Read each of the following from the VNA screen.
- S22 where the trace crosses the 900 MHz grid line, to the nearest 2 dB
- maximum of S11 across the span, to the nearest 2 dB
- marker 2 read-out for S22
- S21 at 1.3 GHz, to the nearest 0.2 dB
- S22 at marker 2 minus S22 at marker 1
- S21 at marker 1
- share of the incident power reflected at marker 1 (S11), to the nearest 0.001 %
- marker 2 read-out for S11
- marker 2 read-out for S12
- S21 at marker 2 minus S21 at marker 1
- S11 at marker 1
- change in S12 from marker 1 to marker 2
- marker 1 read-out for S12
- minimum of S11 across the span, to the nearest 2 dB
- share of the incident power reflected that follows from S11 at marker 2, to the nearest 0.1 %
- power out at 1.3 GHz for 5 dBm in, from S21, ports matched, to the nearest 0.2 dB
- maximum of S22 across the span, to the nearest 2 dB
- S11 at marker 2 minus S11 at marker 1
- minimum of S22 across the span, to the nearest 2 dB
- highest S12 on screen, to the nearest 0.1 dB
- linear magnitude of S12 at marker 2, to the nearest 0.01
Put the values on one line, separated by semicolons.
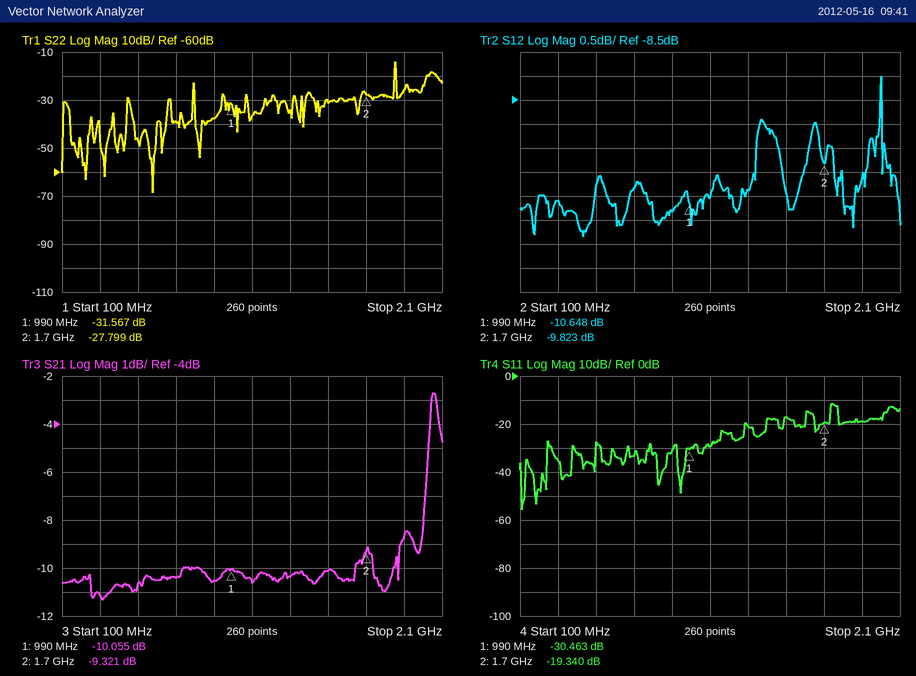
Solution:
-38 dB; -12 dB; -27.799 dB; -10.4 dB; 3.768 dB; -10.055 dB; 0.090 %; -19.340 dB; -9.823 dB; 0.734 dB; -30.463 dB; 0.825 dB; -10.648 dB; -56 dB; 1.2 %; -5.4 dBm; -14 dB; 11.123 dB; -68 dB; -8.0 dB; 0.32
